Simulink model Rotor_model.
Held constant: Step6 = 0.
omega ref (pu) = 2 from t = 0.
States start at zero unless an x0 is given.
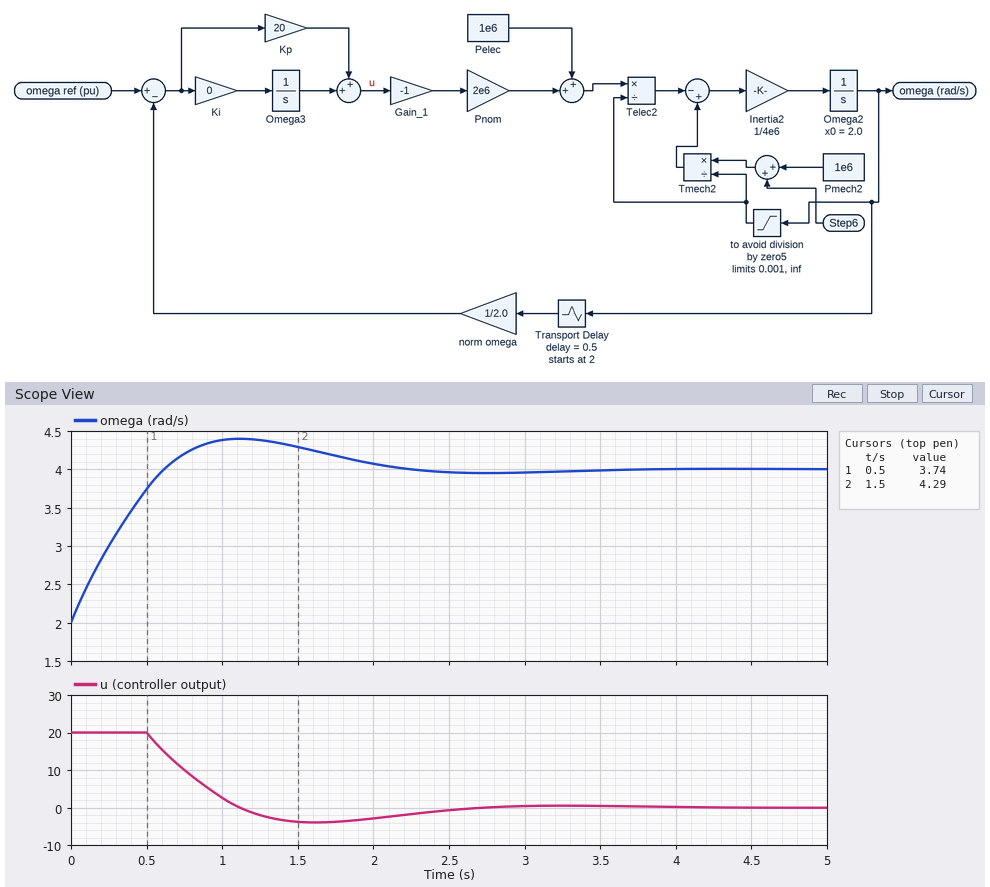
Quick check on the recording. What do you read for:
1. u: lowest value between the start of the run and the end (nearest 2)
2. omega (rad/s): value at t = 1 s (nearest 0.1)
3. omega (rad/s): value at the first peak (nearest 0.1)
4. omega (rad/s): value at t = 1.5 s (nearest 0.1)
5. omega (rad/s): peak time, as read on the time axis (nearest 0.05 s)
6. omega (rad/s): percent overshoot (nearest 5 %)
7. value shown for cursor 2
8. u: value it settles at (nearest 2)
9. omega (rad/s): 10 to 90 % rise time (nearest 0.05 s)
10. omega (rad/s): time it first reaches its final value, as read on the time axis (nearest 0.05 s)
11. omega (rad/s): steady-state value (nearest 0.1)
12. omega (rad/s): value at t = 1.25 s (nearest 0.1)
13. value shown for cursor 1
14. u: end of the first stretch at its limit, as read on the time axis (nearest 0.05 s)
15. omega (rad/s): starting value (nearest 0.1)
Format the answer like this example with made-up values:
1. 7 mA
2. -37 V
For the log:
1. -4
2. 4.4
3. 4.4
4. 4.3
5. 1.10 s
6. 20 %
7. 4.29
8. 0
9. 0.50 s
10. 0.60 s
11. 4.0
12. 4.4
13. 3.74
14. 0.50 s
15. 2.0
